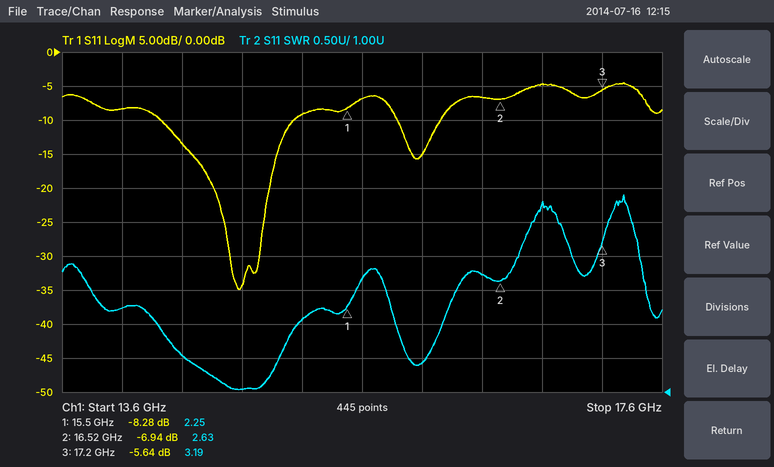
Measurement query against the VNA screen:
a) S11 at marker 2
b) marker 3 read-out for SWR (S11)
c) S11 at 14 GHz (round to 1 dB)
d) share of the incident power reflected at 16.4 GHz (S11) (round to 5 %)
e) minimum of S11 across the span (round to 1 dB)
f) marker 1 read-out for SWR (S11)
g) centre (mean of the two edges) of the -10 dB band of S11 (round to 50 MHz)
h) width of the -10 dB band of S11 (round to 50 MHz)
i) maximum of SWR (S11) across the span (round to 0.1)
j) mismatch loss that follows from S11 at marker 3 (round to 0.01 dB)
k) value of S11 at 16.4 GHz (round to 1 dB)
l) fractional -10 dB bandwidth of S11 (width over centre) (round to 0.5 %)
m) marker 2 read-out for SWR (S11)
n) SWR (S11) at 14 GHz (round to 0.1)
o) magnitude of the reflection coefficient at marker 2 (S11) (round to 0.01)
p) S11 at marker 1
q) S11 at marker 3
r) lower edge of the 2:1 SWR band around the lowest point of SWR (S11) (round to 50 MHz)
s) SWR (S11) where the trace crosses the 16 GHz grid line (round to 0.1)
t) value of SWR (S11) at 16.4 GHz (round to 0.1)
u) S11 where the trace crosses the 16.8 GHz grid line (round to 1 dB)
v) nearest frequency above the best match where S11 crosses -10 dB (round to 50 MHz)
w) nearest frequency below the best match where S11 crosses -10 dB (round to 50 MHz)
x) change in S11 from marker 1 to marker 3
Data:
-6.94 dB
3.19
-8 dB
20 %
-35 dB
2.25
14.70 GHz
900 MHz
3.9
1.38 dB
-7 dB
6.0 %
2.63
2.2
0.45
-8.28 dB
-5.64 dB
14.25 GHz
1.4
2.7
-5 dB
15.15 GHz
14.25 GHz
2.64 dB
